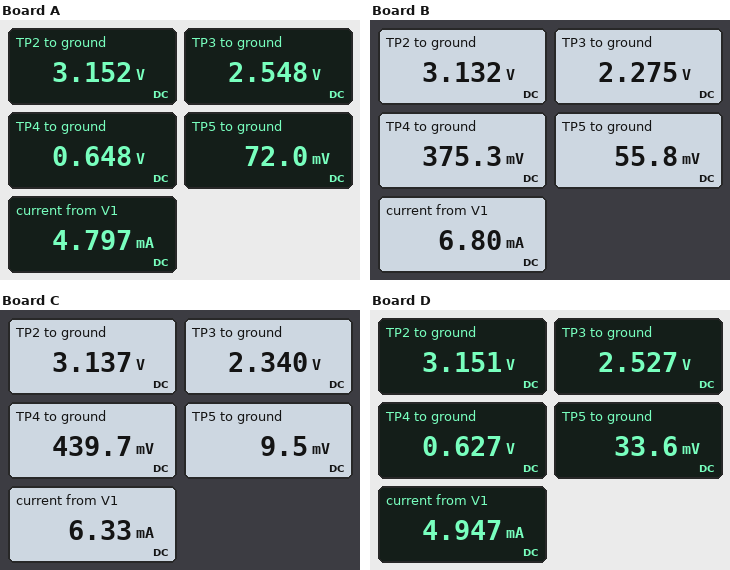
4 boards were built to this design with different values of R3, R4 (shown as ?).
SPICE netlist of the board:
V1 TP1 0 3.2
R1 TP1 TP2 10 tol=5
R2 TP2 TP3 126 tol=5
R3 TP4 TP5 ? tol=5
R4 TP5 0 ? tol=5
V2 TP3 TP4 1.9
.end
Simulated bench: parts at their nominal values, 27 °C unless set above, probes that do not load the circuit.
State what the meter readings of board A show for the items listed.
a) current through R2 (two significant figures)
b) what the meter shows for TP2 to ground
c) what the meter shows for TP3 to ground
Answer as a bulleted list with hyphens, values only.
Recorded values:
- 4.8 mA
- 3.152 V
- 2.548 V
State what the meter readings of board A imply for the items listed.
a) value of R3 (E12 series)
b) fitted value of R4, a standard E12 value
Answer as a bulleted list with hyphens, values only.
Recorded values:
- 120 Ω
- 15 Ω
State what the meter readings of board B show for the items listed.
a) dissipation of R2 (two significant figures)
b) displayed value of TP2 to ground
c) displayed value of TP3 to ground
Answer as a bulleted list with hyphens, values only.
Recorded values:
- 5.8 mW
- 3.132 V
- 2.275 V
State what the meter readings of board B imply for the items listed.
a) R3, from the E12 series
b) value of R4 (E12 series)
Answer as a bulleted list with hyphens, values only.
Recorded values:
- 47 Ω
- 8.2 Ω
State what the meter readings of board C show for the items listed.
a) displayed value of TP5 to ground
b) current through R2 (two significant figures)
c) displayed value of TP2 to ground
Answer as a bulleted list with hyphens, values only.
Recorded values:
- 9.5 mV
- 6.3 mA
- 3.137 V
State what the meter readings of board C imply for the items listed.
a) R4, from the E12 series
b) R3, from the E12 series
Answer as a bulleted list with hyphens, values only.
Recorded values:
- 1.5 Ω
- 68 Ω
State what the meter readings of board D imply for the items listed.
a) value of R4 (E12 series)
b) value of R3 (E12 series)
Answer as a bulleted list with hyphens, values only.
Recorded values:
- 6.8 Ω
- 120 Ω
